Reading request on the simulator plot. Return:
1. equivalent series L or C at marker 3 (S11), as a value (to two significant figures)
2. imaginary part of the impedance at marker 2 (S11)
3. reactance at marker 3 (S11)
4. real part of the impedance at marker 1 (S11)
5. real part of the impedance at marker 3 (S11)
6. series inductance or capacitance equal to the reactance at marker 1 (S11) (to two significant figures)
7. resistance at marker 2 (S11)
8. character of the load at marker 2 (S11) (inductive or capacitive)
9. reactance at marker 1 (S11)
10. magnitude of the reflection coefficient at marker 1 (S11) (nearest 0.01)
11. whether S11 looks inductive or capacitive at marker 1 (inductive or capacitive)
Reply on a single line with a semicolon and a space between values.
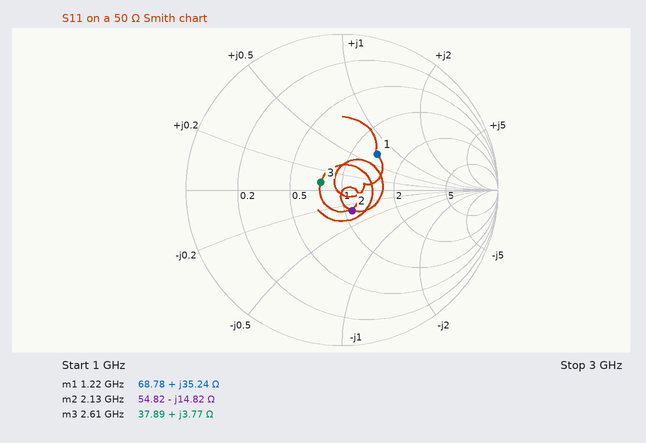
230 pH; -14.82 Ω; +3.77 Ω; 68.78 Ω; 37.89 Ω; 4.6 nH; 54.82 Ω; capacitive; +35.24 Ω; 0.32; inductive
